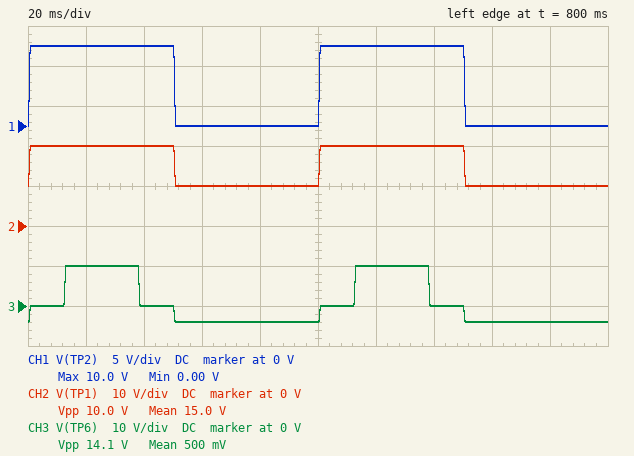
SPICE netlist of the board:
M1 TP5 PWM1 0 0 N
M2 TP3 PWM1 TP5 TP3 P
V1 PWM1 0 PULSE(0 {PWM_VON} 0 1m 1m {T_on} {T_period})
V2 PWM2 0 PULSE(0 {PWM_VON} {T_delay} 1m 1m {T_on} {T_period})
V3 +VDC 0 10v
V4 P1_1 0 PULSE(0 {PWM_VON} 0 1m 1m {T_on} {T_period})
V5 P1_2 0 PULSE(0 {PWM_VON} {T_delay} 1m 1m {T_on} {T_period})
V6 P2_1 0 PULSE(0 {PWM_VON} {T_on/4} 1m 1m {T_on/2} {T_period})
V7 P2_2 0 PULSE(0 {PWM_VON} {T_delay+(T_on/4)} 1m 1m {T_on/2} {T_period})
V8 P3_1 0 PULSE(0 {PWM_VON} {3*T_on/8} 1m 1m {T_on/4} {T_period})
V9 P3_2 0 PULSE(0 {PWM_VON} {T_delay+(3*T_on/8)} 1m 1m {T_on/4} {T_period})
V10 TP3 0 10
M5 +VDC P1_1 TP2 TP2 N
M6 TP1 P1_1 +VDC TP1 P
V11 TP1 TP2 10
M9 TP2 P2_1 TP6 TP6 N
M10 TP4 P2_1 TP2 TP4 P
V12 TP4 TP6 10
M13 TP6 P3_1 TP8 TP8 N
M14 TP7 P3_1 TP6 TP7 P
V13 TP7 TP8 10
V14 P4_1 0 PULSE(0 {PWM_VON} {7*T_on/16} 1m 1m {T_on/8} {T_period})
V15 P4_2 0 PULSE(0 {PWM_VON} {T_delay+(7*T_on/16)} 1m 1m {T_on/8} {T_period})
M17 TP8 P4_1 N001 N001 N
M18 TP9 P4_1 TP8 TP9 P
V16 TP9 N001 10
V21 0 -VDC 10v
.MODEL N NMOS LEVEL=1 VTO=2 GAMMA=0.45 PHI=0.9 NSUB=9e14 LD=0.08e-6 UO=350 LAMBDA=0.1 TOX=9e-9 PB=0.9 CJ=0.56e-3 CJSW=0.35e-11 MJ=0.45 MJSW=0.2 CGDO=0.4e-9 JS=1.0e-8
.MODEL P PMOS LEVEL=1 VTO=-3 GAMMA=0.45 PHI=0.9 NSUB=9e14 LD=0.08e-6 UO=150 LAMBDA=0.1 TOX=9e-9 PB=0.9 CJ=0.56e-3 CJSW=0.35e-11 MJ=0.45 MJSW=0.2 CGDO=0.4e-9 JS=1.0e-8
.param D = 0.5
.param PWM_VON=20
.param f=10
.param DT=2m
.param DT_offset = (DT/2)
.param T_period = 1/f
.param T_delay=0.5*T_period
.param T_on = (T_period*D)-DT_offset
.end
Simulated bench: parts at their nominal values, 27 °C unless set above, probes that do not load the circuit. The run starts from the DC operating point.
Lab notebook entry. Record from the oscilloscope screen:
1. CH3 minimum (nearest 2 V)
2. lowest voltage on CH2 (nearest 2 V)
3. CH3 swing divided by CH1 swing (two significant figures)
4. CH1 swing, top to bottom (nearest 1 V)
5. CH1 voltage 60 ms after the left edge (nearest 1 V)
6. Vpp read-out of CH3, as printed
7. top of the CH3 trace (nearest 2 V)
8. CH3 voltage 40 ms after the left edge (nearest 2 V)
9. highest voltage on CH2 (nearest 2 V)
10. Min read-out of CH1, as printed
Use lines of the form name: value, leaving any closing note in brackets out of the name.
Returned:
CH3 minimum: -4 V
lowest voltage on CH2: 10 V
CH3 swing divided by CH1 swing: 1.4
CH1 swing, top to bottom: 10 V
CH1 voltage 60 ms after the left edge: 0 V
Vpp read-out of CH3, as printed: 14.1 V
top of the CH3 trace: 10 V
CH3 voltage 40 ms after the left edge: 0 V
highest voltage on CH2: 20 V
Min read-out of CH1, as printed: 0.00 V
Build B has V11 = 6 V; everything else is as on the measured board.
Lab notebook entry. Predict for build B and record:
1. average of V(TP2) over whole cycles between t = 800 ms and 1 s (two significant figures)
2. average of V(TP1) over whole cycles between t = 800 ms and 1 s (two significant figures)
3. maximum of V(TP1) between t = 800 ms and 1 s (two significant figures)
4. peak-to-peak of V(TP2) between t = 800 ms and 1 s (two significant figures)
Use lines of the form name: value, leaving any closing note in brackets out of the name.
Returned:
average of V(TP2) over whole cycles between t = 800 ms and 1 s: 7.0 V
average of V(TP1) over whole cycles between t = 800 ms and 1 s: 13 V
maximum of V(TP1) between t = 800 ms and 1 s: 16 V
peak-to-peak of V(TP2) between t = 800 ms and 1 s: 6.0 V
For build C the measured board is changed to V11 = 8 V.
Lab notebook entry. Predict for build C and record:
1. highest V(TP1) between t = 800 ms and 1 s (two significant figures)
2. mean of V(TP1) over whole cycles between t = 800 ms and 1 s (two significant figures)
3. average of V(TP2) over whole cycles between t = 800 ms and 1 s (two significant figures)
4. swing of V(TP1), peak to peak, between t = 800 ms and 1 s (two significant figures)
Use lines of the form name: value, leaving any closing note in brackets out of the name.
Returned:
highest V(TP1) between t = 800 ms and 1 s: 18 V
mean of V(TP1) over whole cycles between t = 800 ms and 1 s: 14 V
average of V(TP2) over whole cycles between t = 800 ms and 1 s: 6.0 V
swing of V(TP1), peak to peak, between t = 800 ms and 1 s: 8.0 V
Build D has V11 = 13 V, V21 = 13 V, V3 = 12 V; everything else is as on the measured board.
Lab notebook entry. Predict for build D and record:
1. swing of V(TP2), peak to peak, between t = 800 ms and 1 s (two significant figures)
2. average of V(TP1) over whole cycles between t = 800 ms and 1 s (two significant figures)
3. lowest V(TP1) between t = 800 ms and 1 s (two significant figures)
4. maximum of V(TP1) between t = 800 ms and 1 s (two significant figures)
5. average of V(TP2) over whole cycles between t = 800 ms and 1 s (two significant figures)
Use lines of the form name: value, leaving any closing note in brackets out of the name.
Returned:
swing of V(TP2), peak to peak, between t = 800 ms and 1 s: 13 V
average of V(TP1) over whole cycles between t = 800 ms and 1 s: 18 V
lowest V(TP1) between t = 800 ms and 1 s: 12 V
maximum of V(TP1) between t = 800 ms and 1 s: 25 V
average of V(TP2) over whole cycles between t = 800 ms and 1 s: 5.4 V
